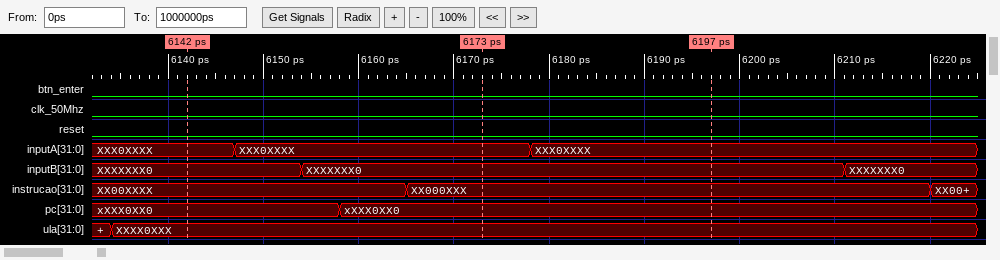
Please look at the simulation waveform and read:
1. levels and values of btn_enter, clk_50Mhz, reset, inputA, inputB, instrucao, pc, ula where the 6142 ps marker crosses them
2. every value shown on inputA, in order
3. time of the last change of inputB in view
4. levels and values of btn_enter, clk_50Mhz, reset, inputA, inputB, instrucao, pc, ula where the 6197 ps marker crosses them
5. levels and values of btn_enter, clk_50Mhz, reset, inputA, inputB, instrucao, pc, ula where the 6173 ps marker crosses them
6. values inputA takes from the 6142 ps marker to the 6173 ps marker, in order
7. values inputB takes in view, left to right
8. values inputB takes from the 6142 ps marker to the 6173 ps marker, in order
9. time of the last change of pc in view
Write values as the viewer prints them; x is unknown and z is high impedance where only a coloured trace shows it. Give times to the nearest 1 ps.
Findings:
btn_enter=0, clk_50Mhz=0, reset=0, inputA=XXX0XXXX, inputB=XXXXXXX0, instrucao=XX00XXXX, pc=xXXX0XX0, ula=XXXX0XXX
XXX0XXXX, XXX0XXXX, XXX0XXXX
6211 ps
btn_enter=0, clk_50Mhz=0, reset=0, inputA=XXX0XXXX, inputB=XXXXXXX0, instrucao=XX000XXX, pc=xXXX0XX0, ula=XXXX0XXX
btn_enter=0, clk_50Mhz=0, reset=0, inputA=XXX0XXXX, inputB=XXXXXXX0, instrucao=XX000XXX, pc=xXXX0XX0, ula=XXXX0XXX
XXX0XXXX, XXX0XXXX
XXXXXXX0, XXXXXXX0, XXXXXXX0
XXXXXXX0, XXXXXXX0
6158 ps
